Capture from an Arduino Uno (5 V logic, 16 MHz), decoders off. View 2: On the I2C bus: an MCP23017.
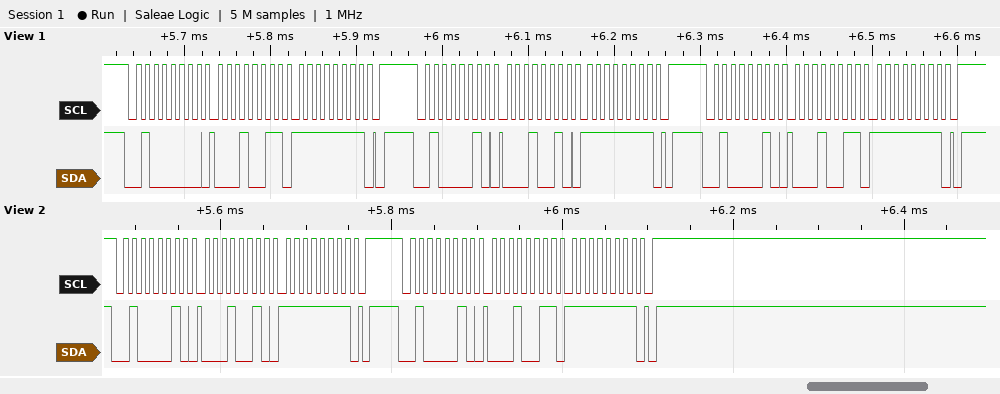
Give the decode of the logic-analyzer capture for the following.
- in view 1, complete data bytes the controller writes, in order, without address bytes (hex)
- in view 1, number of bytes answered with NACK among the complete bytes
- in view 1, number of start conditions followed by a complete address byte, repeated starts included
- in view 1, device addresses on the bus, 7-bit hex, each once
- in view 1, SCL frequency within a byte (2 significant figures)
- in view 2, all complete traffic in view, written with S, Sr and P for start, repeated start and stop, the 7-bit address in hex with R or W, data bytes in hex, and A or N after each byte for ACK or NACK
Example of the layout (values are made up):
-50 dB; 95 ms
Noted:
13 FF 12 FF 13 FF; 0; 3; 0x20 0x21; 100 kHz; S 21W A 12 A FF A P S 21W A 13 A FF A P
